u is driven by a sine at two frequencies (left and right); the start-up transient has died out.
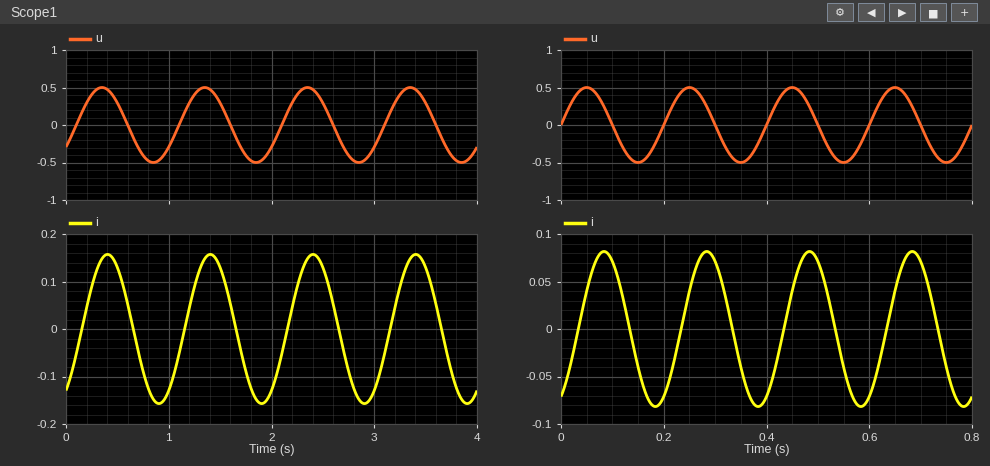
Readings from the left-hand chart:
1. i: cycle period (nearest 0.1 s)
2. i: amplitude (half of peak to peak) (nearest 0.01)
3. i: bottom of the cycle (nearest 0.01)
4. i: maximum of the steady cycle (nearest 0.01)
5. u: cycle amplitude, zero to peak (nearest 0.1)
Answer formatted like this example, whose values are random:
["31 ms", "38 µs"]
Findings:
["1.0 s", "0.16", "-0.16", "0.16", "0.5"]
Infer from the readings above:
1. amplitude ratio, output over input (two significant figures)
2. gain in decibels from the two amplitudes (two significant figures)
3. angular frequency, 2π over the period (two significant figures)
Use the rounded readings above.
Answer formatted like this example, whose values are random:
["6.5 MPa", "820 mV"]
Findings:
["0.32", "-9.9 dB", "6.3 rad/s"]
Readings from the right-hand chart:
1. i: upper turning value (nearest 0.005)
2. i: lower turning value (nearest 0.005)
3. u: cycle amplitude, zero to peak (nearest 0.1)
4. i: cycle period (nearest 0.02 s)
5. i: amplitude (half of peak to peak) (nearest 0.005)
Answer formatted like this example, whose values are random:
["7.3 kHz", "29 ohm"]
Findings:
["0.080", "-0.080", "0.5", "0.20 s", "0.080"]
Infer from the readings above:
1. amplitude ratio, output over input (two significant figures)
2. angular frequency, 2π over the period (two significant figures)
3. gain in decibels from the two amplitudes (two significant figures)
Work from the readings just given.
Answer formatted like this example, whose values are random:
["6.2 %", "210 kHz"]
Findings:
["0.16", "31 rad/s", "-16 dB"]
